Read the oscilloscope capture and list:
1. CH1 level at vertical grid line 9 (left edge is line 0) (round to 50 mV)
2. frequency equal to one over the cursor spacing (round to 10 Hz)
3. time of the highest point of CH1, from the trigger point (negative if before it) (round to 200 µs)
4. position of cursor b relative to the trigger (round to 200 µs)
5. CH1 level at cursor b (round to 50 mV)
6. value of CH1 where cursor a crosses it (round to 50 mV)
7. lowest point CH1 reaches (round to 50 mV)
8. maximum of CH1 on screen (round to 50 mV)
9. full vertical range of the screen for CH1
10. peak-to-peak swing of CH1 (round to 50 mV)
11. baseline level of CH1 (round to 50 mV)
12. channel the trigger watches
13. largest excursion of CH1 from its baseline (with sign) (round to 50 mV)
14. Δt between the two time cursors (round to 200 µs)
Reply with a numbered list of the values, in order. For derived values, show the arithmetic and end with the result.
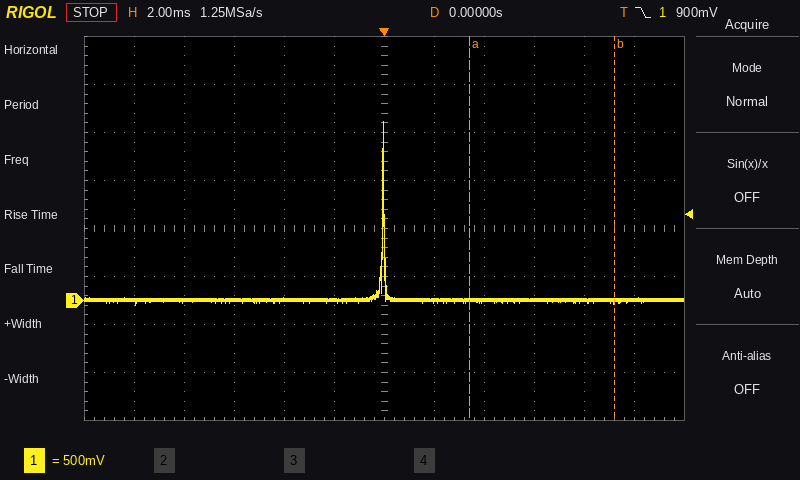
1. 0 mV
2. 1 / 5.8 ms ≈ 170 Hz
3. 0.0 ms
4. +9.2 ms
5. 0 mV
6. 0 mV
7. -50 mV
8. 1.85 V
9. 4 V
10. 1.85 V − (-50 mV) = 1.90 V
11. 0 mV
12. CH1
13. 1.85 V − (0 mV) = +1.85 V
14. 5.8 ms
